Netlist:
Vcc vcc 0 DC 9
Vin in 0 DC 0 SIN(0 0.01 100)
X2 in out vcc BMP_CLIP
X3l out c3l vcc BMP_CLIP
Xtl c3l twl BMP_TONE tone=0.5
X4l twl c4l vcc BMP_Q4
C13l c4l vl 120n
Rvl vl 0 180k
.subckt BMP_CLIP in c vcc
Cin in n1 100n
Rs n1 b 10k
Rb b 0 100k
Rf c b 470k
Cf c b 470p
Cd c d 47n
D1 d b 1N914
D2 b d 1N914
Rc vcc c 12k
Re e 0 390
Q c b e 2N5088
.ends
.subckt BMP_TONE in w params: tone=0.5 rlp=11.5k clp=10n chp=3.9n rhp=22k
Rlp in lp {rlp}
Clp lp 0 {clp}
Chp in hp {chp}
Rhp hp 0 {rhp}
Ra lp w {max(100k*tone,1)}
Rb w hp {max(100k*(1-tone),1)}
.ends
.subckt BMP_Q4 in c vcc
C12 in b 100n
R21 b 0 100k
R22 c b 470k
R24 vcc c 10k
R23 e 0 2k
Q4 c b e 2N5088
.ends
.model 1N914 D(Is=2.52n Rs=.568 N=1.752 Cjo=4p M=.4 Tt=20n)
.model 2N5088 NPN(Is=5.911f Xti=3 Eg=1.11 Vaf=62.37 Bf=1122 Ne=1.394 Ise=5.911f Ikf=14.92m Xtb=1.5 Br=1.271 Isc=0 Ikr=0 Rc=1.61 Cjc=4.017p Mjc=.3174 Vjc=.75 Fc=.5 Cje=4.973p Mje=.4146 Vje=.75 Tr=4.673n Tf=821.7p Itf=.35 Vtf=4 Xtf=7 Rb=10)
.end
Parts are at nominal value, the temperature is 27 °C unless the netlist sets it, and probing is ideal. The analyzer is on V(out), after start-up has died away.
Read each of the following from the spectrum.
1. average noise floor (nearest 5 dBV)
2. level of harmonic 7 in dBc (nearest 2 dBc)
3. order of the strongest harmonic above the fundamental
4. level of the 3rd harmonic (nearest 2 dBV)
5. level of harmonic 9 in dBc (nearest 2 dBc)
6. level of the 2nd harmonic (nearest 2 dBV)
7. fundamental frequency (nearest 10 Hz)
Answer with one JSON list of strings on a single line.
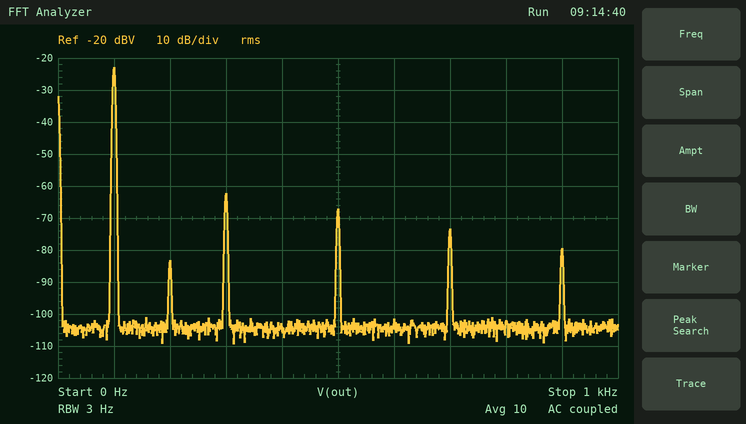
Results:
["-105 dBV", "-50 dBc", "3", "-62 dBV", "-56 dBc", "-84 dBV", "100 Hz"]
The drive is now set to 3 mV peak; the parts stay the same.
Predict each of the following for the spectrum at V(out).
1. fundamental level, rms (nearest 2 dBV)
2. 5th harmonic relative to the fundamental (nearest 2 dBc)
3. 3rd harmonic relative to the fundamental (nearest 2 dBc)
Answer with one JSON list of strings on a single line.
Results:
["-34 dBV", "-56 dBc", "-38 dBc"]
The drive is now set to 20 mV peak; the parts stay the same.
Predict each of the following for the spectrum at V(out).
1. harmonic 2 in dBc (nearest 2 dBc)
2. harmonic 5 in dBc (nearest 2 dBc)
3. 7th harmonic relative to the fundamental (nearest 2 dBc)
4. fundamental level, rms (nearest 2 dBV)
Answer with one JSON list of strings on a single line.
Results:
["-56 dBc", "-46 dBc", "-52 dBc", "-18 dBV"]
